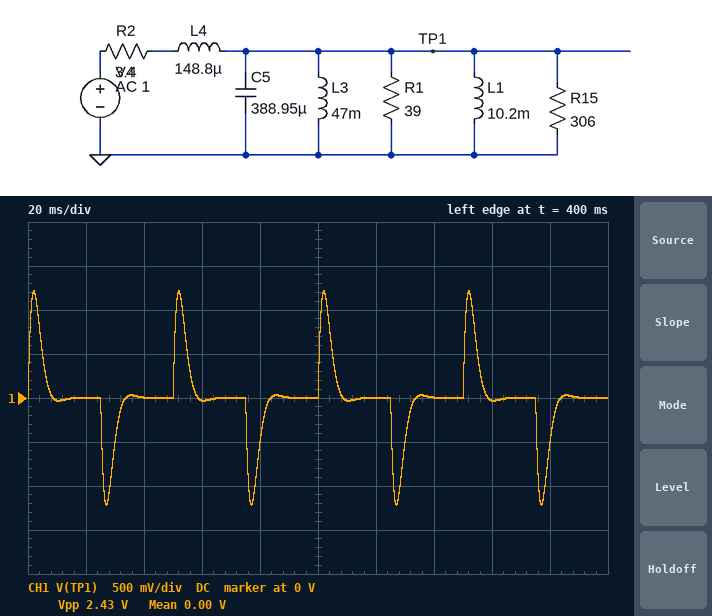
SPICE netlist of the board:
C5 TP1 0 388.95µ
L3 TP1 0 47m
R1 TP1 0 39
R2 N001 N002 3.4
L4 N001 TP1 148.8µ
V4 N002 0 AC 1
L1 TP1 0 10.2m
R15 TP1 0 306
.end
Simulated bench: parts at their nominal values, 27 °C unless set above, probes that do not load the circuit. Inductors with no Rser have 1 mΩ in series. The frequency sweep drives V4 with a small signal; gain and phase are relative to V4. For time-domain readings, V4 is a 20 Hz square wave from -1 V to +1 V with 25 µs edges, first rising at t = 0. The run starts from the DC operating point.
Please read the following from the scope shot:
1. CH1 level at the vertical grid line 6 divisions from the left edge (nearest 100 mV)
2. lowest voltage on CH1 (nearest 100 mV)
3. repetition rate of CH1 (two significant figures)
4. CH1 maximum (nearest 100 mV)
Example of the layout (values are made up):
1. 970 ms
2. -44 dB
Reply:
1. 0 V
2. -1.2 V
3. 20 Hz
4. 1.2 V
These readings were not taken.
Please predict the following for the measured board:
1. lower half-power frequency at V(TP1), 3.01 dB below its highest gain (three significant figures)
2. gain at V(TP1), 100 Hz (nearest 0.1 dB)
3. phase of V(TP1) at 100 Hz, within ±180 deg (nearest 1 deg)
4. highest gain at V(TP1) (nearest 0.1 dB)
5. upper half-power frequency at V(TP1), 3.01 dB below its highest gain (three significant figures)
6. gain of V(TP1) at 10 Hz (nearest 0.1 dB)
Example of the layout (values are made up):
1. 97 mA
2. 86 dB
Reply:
1. 44.4 Hz
2. -0.9 dB
3. -10 deg
4. -0.8 dB
5. 181 Hz
6. -16.2 dB
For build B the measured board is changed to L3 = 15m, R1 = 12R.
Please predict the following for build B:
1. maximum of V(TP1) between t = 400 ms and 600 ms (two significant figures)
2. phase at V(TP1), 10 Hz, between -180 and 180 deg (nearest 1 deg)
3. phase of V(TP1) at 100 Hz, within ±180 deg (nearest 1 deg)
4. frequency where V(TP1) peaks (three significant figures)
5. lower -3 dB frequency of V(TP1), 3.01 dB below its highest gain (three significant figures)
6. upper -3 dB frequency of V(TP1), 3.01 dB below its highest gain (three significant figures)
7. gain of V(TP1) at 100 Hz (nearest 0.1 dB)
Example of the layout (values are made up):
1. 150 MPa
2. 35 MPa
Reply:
1. 1.0 V
2. 81 deg
3. 2 deg
4. 105 Hz
5. 52.1 Hz
6. 213 Hz
7. -2.3 dB
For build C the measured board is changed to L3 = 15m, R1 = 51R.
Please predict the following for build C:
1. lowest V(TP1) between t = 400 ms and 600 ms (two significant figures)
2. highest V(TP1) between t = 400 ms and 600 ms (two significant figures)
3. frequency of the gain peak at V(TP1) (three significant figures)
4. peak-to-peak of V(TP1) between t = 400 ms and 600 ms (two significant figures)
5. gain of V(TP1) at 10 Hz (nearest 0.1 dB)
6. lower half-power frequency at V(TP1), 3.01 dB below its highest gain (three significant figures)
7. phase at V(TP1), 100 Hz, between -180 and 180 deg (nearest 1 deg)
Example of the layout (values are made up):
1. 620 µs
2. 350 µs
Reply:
1. -1.1 V
2. 1.1 V
3. 105 Hz
4. 2.3 V
5. -19.0 dB
6. 57.8 Hz
7. 3 deg
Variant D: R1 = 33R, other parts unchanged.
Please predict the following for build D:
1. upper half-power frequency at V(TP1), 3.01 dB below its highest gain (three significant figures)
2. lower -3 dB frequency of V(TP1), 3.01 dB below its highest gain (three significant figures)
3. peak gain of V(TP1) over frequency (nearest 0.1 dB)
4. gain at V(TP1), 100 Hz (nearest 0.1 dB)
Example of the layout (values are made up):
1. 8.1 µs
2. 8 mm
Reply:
1. 183 Hz
2. 44.0 Hz
3. -0.9 dB
4. -1.0 dB
